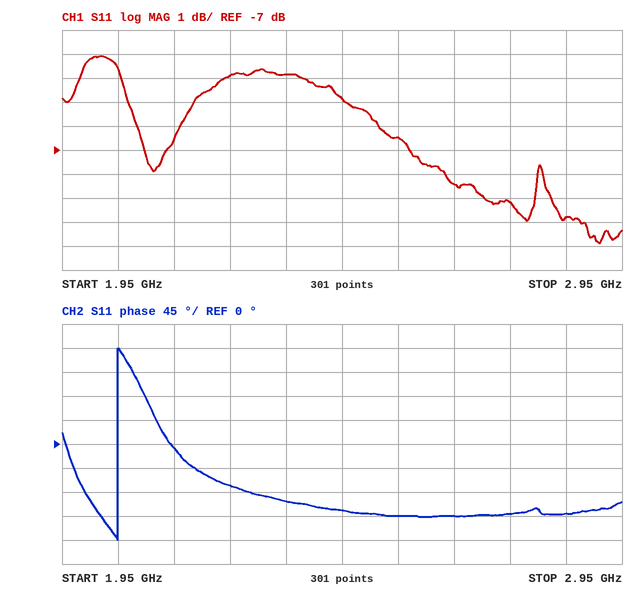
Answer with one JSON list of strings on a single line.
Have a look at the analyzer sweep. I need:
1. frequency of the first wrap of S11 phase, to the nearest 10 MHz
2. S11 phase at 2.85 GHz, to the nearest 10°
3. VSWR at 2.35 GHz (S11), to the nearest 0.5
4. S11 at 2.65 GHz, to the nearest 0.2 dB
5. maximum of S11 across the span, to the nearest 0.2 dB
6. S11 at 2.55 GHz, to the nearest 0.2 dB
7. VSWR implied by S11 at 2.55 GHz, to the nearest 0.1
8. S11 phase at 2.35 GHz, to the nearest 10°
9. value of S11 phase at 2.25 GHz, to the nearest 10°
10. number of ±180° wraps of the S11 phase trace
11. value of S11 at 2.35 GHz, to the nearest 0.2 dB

["2.05 GHz", "-130°", "4.5", "-8.4 dB", "-3.0 dB", "-6.4 dB", "2.8", "-110°", "-80°", "1", "-3.8 dB"]
